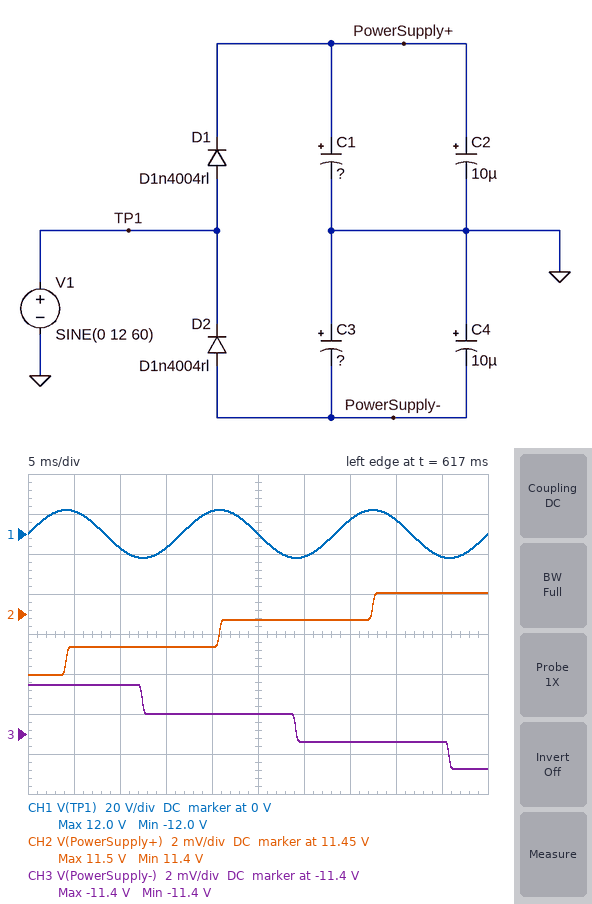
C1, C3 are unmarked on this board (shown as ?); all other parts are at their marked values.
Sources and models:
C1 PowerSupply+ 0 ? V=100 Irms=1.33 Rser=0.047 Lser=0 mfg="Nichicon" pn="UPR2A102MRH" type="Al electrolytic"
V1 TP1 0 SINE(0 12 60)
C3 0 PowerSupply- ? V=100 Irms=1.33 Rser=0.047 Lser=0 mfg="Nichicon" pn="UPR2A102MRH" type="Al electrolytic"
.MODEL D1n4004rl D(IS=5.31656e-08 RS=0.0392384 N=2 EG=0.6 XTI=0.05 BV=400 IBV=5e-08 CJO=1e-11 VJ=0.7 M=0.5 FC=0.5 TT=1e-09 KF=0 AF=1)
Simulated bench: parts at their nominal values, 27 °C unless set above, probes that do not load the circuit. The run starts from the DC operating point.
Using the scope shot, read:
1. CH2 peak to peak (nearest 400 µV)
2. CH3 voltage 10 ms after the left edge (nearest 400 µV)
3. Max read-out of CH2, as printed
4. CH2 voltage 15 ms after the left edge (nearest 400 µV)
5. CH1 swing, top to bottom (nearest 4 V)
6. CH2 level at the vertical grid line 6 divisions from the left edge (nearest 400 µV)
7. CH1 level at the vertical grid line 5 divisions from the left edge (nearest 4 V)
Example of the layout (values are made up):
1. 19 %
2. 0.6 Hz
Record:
1. 4.0 mV
2. -11.3976 V
3. 11.5 V
4. 11.4504 V
5. 24 V
6. 11.4516 V
7. 0 V
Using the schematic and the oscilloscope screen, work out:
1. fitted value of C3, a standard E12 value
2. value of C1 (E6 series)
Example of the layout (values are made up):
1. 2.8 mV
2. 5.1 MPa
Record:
1. 1.8 mF
2. 680 µF
